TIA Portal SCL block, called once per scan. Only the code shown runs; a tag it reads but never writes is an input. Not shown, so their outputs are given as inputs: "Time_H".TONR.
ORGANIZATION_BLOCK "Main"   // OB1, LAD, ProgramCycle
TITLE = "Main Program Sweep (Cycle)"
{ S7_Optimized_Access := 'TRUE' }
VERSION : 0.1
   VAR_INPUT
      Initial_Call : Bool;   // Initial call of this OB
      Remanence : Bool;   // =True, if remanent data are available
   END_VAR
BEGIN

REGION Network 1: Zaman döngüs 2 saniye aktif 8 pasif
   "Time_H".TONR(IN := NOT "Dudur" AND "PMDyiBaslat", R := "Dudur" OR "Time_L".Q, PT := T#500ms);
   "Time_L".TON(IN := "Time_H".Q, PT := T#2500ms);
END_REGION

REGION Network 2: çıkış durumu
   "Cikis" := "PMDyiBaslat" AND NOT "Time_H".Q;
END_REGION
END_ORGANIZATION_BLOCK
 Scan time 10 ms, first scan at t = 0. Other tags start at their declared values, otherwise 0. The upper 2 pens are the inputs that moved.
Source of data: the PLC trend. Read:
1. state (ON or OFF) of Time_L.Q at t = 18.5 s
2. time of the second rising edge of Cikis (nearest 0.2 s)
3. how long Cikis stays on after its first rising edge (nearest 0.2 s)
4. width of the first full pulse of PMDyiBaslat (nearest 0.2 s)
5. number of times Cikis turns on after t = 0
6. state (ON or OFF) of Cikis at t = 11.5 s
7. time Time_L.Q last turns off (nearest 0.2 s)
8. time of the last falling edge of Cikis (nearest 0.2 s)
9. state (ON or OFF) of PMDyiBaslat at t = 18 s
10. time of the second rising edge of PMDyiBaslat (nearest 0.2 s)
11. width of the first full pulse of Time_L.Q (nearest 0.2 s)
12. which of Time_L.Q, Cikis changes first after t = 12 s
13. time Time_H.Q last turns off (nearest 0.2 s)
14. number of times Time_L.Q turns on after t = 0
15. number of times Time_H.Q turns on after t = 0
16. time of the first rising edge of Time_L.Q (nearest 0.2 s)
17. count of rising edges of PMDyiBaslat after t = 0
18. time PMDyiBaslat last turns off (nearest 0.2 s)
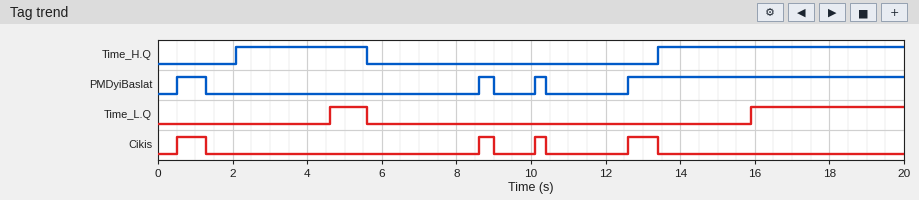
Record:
ON
8.6 s
0.8 s
0.8 s
4
OFF
5.6 s
13.4 s
ON
8.6 s
1.0 s
Cikis
5.6 s
2
2
4.6 s
4
10.4 s
